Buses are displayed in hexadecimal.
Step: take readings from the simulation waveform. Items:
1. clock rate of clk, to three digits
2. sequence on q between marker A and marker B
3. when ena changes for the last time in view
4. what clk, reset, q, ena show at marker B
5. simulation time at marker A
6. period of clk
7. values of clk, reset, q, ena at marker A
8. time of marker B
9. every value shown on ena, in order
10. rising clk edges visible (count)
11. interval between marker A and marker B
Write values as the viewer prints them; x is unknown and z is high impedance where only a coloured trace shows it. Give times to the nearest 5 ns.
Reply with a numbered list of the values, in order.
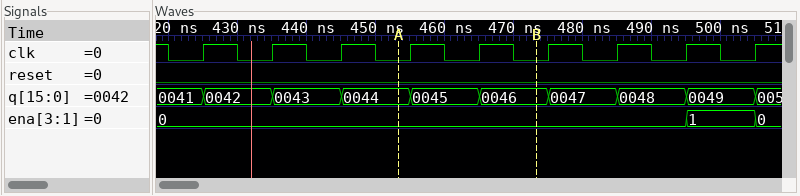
1. 100 MHz
2. 0044, 0045, 0046
3. 505 ns
4. clk=0, reset=0, q=0046, ena=0
5. 455 ns
6. 10 ns
7. clk=0, reset=0, q=0044, ena=0
8. 475 ns
9. 0, 1, 0
10. 9
11. 20 ns
